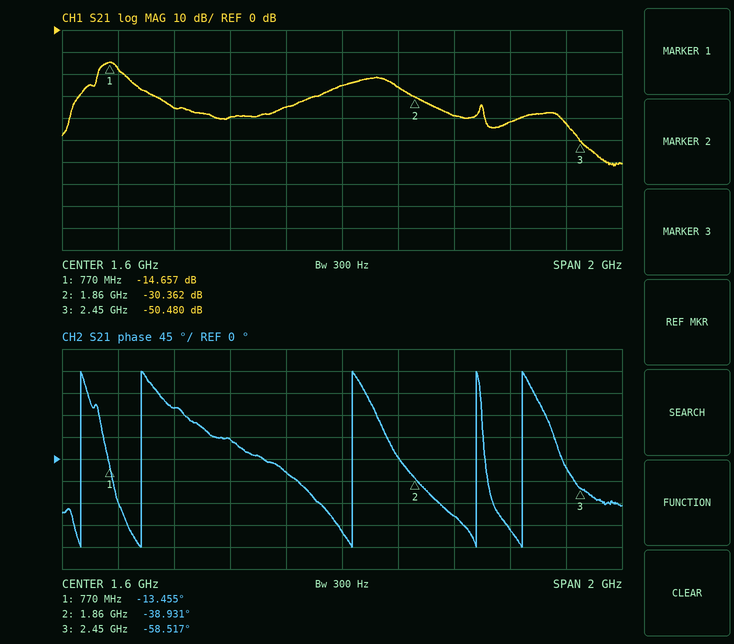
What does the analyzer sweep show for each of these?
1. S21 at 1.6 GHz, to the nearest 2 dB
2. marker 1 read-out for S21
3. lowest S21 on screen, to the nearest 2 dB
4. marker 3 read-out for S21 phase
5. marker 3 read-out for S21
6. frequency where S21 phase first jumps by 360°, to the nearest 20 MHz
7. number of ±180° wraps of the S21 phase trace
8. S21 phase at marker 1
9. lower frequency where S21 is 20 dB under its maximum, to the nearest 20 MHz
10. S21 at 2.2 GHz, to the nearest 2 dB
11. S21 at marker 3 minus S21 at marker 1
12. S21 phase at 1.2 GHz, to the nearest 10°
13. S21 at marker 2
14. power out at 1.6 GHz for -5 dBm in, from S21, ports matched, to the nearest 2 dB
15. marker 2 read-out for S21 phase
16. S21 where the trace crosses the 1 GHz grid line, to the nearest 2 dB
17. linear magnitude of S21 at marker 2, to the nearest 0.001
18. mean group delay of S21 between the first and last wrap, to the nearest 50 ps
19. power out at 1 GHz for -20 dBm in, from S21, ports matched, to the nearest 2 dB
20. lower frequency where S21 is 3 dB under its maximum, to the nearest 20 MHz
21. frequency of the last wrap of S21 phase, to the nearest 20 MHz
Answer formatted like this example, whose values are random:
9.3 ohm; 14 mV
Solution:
-26 dB; -14.657 dB; -62 dB; -58.517°; -50.480 dB; 660 MHz; 5; -13.455°; 640 MHz; -42 dB; -35.823 dB; 40°; -30.362 dB; -30 dBm; -38.931°; -36 dB; 0.030; 2.55 ns; -56 dBm; 740 MHz; 2.24 GHz
